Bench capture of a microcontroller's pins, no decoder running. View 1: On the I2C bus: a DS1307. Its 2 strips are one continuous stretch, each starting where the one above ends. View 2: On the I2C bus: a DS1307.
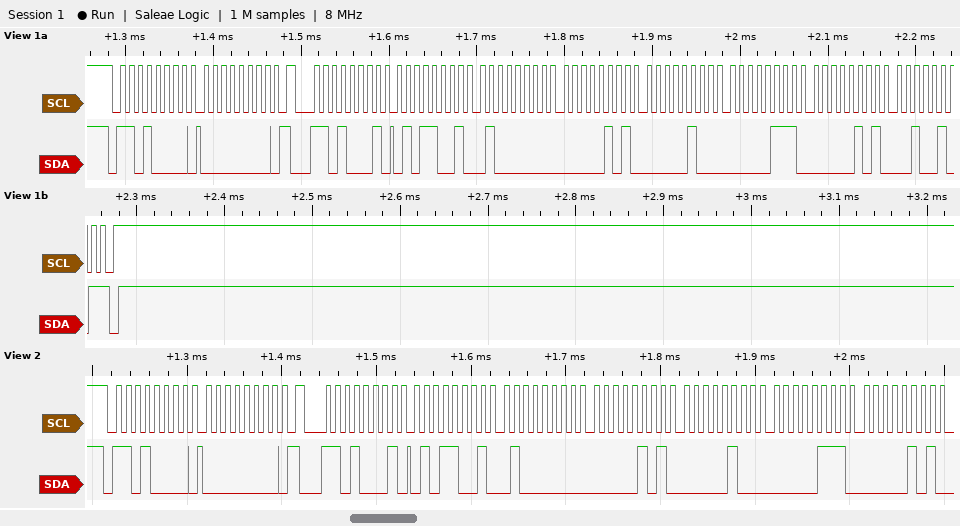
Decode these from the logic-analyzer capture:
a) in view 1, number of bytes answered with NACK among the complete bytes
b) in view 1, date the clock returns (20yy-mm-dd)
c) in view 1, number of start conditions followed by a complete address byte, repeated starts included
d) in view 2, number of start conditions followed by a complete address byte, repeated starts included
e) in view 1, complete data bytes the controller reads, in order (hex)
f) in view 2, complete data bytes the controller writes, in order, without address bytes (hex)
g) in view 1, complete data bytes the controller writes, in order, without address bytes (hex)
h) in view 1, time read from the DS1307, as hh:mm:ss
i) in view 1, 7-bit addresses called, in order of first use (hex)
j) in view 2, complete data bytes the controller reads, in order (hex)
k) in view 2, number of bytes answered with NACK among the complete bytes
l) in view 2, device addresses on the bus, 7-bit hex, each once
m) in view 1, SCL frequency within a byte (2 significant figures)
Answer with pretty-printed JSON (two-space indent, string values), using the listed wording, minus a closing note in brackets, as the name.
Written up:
{
  "in view 1, number of bytes answered with NACK among the complete bytes": "1",
  "in view 1, date the clock returns": "2025-05-07",
  "in view 1, number of start conditions followed by a complete address byte, repeated starts included": "2",
  "in view 2, number of start conditions followed by a complete address byte, repeated starts included": "2",
  "in view 1, complete data bytes the controller reads, in order": "59 40 05 04 07 05 25",
  "in view 2, complete data bytes the controller writes, in order, without address bytes": "00",
  "in view 1, complete data bytes the controller writes, in order, without address bytes": "00",
  "in view 1, time read from the DS1307, as hh:mm:ss": "05:40:59",
  "in view 1, 7-bit addresses called, in order of first use": "0x68",
  "in view 2, complete data bytes the controller reads, in order": "59 40 05 04 07 05",
  "in view 2, number of bytes answered with NACK among the complete bytes": "0",
  "in view 2, device addresses on the bus, 7-bit hex, each once": "0x68",
  "in view 1, SCL frequency within a byte": "100 kHz"
}
